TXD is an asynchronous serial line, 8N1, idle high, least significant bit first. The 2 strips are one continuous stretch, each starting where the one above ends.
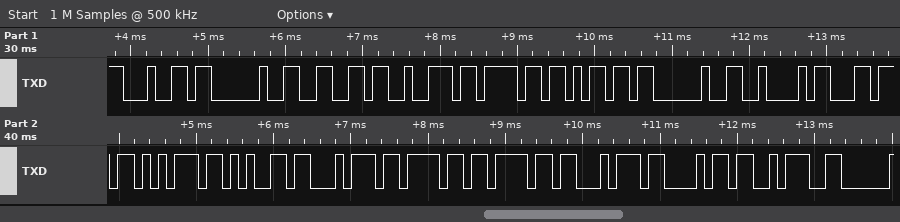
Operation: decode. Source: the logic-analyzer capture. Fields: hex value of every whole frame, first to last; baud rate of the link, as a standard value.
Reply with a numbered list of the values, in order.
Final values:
1. 0x64 0x20 0x66 0x72 0x6F 0x6D 0x20 0x42 0x6C 0x75 0x65 0x74 0x6F 0x6F 0x74 0x68 0x3A
2. 9600 baud
